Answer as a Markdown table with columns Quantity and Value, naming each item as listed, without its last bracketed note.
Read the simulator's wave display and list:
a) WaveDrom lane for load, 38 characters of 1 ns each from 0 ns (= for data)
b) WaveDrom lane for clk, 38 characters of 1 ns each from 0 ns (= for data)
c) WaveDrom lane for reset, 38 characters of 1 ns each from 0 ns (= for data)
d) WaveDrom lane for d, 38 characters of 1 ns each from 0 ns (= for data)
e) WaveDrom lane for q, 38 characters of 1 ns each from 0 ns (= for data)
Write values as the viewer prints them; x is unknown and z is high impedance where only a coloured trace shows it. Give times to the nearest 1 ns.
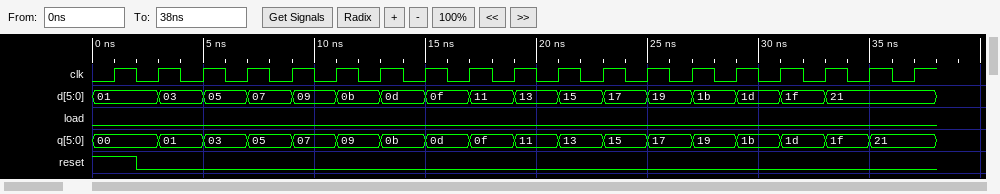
| Quantity | Value |
|---|---|
| WaveDrom lane for load, 38 characters of 1 ns each from 0 ns | {name: 'load', wave: '0.....................................'} |
| WaveDrom lane for clk, 38 characters of 1 ns each from 0 ns | {name: 'clk', wave: '01010101010101010101010101010101010101'} |
| WaveDrom lane for reset, 38 characters of 1 ns each from 0 ns | {name: 'reset', wave: '1.0...................................'} |
| WaveDrom lane for d, 38 characters of 1 ns each from 0 ns | {name: 'd', wave: '=..=.=.=.=.=.=.=.=.=.=.=.=.=.=.=.=....', data: '01 03 05 07 09 0b 0d 0f 11 13 15 17 19 1b 1d 1f 21'} |
| WaveDrom lane for q, 38 characters of 1 ns each from 0 ns | {name: 'q', wave: '=..=.=.=.=.=.=.=.=.=.=.=.=.=.=.=.=.=..', data: '00 01 03 05 07 09 0b 0d 0f 11 13 15 17 19 1b 1d 1f 21'} |
